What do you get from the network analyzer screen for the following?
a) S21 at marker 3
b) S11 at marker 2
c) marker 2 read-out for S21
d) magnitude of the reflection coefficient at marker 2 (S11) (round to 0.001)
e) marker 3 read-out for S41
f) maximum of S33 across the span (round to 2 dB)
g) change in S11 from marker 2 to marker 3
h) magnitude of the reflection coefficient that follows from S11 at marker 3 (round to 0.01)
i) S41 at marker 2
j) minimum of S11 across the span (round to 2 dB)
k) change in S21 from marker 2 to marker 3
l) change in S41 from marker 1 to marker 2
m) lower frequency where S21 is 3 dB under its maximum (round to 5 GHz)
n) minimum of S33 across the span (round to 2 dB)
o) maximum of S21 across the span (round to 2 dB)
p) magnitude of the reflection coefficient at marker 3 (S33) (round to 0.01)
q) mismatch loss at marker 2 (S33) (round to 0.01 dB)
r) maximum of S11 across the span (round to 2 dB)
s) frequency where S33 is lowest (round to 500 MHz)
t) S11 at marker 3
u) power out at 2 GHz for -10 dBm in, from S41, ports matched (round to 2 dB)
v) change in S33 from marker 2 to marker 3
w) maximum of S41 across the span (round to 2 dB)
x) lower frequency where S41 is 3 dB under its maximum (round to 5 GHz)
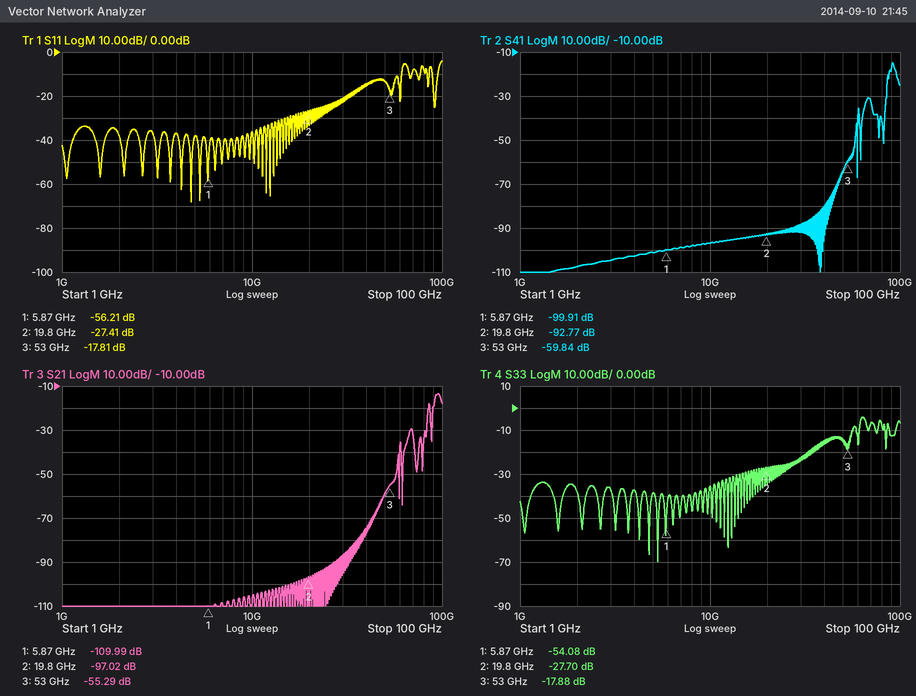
-55.29 dB
-27.41 dB
-97.02 dB
0.043
-59.84 dB
-4 dB
9.60 dB
0.13
-92.77 dB
-68 dB
41.73 dB
7.14 dB
90 GHz
-70 dB
-14 dB
0.13
0.01 dB
-4 dB
5.5 GHz
-17.81 dB
-118 dBm
9.82 dB
-14 dB
90 GHz
